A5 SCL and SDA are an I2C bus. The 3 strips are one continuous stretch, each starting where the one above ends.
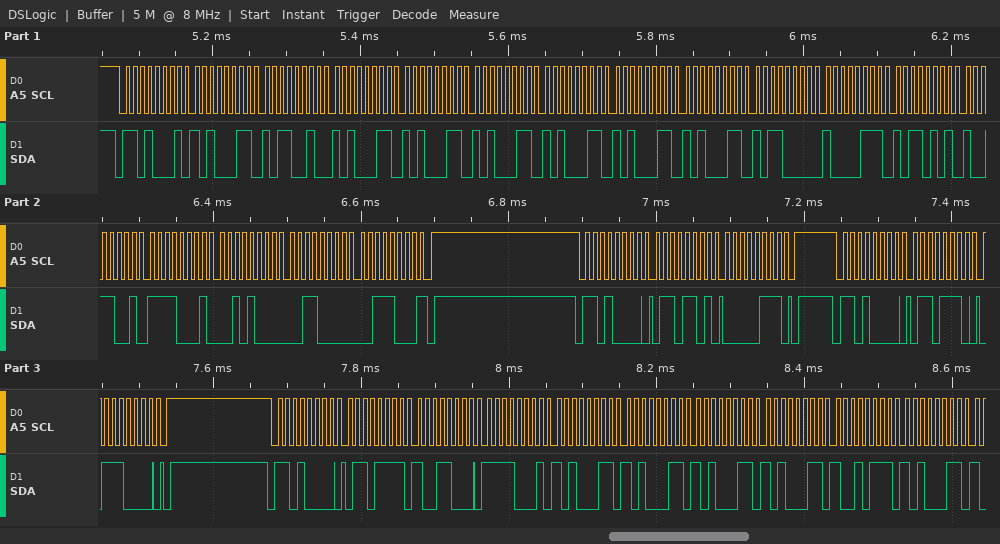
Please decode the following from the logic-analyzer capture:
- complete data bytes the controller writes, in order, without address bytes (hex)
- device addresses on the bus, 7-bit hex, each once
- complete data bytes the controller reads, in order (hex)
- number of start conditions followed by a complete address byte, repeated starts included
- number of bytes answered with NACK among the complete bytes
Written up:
6D 07 6E 70 6F 98 F1 A3 A3 A3 A3 97 A3
0x68
A3 B2 A3 A3 A3 A3 A3 A3 B0 87 B5 99 F1 28 30 38
4
1
